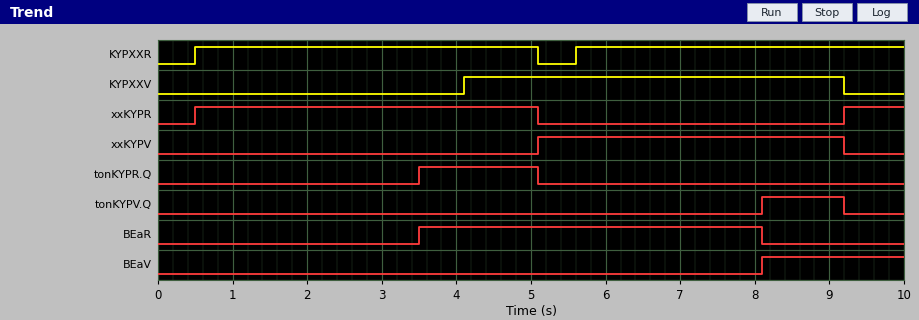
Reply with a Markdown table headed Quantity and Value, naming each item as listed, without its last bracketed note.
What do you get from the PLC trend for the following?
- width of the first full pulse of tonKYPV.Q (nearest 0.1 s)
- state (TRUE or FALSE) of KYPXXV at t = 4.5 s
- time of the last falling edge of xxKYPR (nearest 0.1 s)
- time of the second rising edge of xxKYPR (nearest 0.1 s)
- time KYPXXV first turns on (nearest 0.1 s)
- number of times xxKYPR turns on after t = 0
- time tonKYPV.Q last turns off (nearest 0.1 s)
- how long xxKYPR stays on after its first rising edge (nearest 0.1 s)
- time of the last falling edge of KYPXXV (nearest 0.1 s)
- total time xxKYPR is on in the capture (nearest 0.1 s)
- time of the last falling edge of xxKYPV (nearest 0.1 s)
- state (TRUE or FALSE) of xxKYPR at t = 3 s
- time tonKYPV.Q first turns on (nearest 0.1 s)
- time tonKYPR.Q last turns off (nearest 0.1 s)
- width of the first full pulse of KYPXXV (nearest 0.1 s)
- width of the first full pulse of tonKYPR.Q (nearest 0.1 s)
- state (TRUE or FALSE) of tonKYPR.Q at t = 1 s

| Quantity | Value |
|---|---|
| width of the first full pulse of tonKYPV.Q | 1.1 s |
| state (TRUE or FALSE) of KYPXXV at t = 4.5 s | TRUE |
| time of the last falling edge of xxKYPR | 5.1 s |
| time of the second rising edge of xxKYPR | 9.2 s |
| time KYPXXV first turns on | 4.1 s |
| number of times xxKYPR turns on after t = 0 | 2 |
| time tonKYPV.Q last turns off | 9.2 s |
| how long xxKYPR stays on after its first rising edge | 4.6 s |
| time of the last falling edge of KYPXXV | 9.2 s |
| total time xxKYPR is on in the capture | 5.4 s |
| time of the last falling edge of xxKYPV | 9.2 s |
| state (TRUE or FALSE) of xxKYPR at t = 3 s | TRUE |
| time tonKYPV.Q first turns on | 8.1 s |
| time tonKYPR.Q last turns off | 5.1 s |
| width of the first full pulse of KYPXXV | 5.1 s |
| width of the first full pulse of tonKYPR.Q | 1.6 s |
| state (TRUE or FALSE) of tonKYPR.Q at t = 1 s | FALSE |
